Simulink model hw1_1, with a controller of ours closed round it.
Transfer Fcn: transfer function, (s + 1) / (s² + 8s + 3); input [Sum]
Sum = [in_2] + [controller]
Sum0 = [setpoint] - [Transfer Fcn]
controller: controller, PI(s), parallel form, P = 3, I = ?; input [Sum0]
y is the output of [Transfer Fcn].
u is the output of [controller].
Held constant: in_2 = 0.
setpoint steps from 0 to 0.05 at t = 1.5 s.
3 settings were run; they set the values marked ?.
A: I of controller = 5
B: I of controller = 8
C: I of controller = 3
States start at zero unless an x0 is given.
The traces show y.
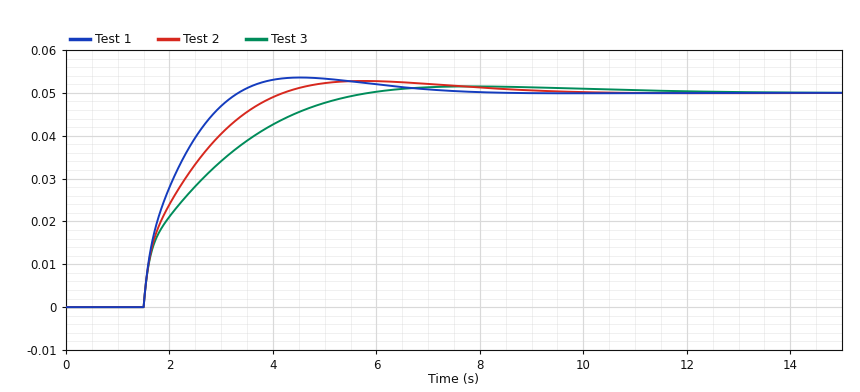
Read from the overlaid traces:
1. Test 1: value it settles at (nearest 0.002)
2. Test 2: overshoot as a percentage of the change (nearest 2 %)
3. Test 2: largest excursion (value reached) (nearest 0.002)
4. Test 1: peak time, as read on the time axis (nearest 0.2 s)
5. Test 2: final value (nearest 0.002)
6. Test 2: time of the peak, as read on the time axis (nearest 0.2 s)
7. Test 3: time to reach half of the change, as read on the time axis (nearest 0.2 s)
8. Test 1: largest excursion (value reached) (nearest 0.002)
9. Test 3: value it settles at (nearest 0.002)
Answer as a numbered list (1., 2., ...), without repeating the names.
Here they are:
1. 0.050
2. 6 %
3. 0.052
4. 4.6 s
5. 0.050
6. 5.8 s
7. 2.2 s
8. 0.054
9. 0.050
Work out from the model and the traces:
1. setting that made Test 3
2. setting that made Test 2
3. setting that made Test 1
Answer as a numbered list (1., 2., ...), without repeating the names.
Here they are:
1. C
2. A
3. B
